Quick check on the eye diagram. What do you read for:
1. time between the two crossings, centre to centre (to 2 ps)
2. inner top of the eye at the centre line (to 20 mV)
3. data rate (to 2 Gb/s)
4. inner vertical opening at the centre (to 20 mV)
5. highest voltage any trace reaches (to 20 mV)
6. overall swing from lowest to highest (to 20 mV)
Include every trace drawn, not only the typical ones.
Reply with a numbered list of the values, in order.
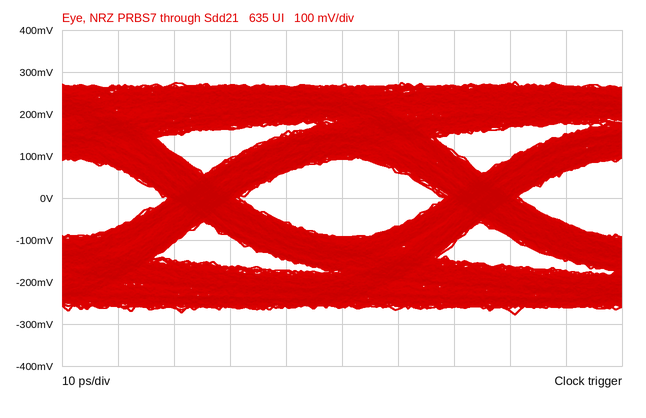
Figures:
1. 50 ps
2. 100 mV
3. 20 Gb/s
4. 180 mV
5. 280 mV
6. 560 mV
